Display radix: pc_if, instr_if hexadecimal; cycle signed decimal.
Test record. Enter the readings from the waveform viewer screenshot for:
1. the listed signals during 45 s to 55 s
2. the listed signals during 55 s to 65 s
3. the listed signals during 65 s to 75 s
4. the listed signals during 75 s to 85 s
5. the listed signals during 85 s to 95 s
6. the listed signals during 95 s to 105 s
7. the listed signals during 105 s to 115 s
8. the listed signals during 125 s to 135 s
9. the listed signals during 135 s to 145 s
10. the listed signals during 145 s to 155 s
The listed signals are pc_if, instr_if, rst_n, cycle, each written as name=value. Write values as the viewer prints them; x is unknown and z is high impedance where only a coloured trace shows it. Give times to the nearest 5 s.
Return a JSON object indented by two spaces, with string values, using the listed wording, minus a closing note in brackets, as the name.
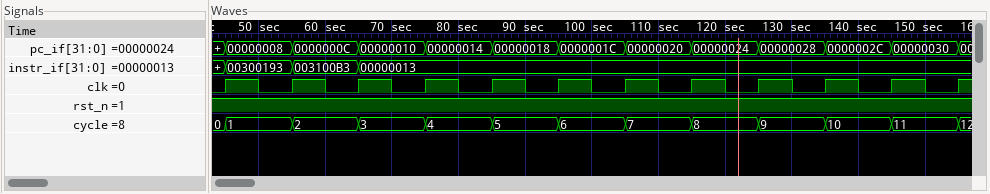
{
  "the listed signals during 45 s to 55 s": "pc_if=00000008, instr_if=00300193, rst_n=1, cycle=1",
  "the listed signals during 55 s to 65 s": "pc_if=0000000C, instr_if=003100B3, rst_n=1, cycle=2",
  "the listed signals during 65 s to 75 s": "pc_if=00000010, instr_if=00000013, rst_n=1, cycle=3",
  "the listed signals during 75 s to 85 s": "pc_if=00000014, instr_if=00000013, rst_n=1, cycle=4",
  "the listed signals during 85 s to 95 s": "pc_if=00000018, instr_if=00000013, rst_n=1, cycle=5",
  "the listed signals during 95 s to 105 s": "pc_if=0000001C, instr_if=00000013, rst_n=1, cycle=6",
  "the listed signals during 105 s to 115 s": "pc_if=00000020, instr_if=00000013, rst_n=1, cycle=7",
  "the listed signals during 125 s to 135 s": "pc_if=00000028, instr_if=00000013, rst_n=1, cycle=9",
  "the listed signals during 135 s to 145 s": "pc_if=0000002C, instr_if=00000013, rst_n=1, cycle=10",
  "the listed signals during 145 s to 155 s": "pc_if=00000030, instr_if=00000013, rst_n=1, cycle=11"
}
